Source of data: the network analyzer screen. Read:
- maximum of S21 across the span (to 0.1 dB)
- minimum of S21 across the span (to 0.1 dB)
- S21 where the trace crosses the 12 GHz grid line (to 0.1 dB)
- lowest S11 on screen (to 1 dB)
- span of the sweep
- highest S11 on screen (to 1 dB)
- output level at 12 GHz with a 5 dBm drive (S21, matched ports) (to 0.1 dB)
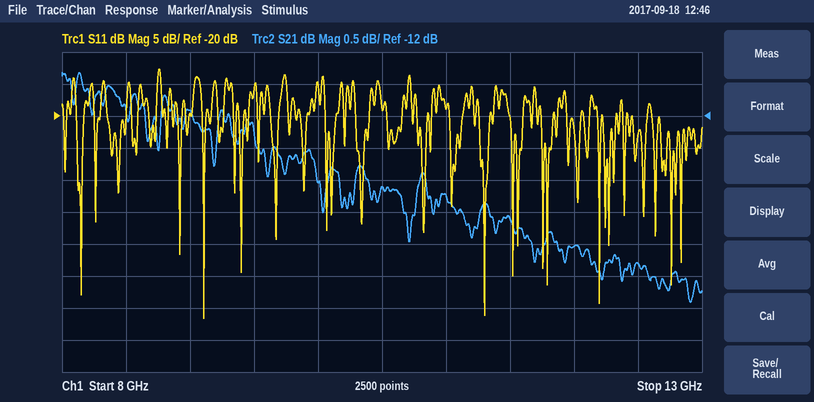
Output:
-11.3 dB
-14.9 dB
-14.0 dB
-52 dB
5 GHz
-13 dB
-9.0 dBm
